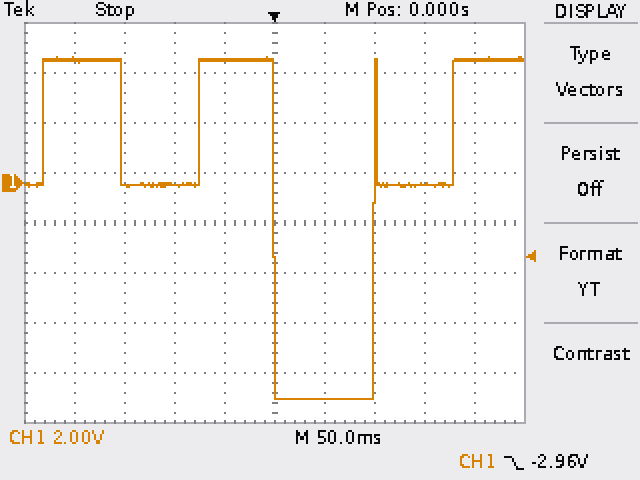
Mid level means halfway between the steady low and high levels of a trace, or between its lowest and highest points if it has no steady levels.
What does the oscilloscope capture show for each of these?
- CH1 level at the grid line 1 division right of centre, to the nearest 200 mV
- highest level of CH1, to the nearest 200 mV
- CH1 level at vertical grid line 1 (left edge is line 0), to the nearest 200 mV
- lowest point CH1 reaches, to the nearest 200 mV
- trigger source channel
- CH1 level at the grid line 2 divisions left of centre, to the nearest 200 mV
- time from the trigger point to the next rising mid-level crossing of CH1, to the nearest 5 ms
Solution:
-8.6 V
5.0 V
5.0 V
-8.6 V
CH1
0.0 V
100 ms
